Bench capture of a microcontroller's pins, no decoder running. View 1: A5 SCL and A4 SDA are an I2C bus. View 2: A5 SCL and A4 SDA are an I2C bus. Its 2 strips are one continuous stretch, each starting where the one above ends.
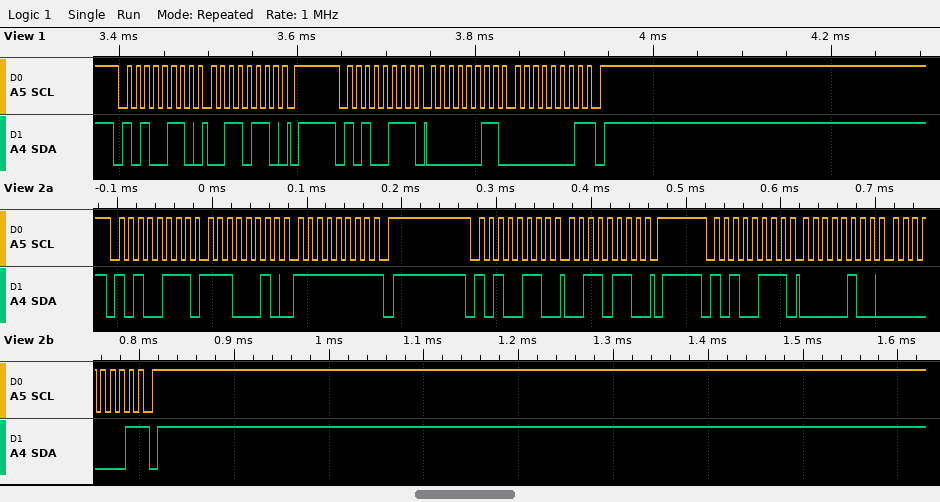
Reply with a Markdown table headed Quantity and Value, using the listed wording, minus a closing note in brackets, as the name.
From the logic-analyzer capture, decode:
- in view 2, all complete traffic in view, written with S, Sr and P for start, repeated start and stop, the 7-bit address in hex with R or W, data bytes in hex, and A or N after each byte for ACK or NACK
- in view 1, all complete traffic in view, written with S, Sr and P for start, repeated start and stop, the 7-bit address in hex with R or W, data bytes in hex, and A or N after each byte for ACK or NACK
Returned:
| Quantity | Value |
|---|---|
| in view 2, all complete traffic in view, written with S, Sr and P for start, repeated start and stop, the 7-bit address in hex with R or W, data bytes in hex, and A or N after each byte for ACK or NACK | S 53R A E2 A FF N P S 53W A 36 A P S 53R A 04 A 01 N P |
| in view 1, all complete traffic in view, written with S, Sr and P for start, repeated start and stop, the 7-bit address in hex with R or W, data bytes in hex, and A or N after each byte for ACK or NACK | S 53W A 36 A P S 53R A 03 A 01 N P |
